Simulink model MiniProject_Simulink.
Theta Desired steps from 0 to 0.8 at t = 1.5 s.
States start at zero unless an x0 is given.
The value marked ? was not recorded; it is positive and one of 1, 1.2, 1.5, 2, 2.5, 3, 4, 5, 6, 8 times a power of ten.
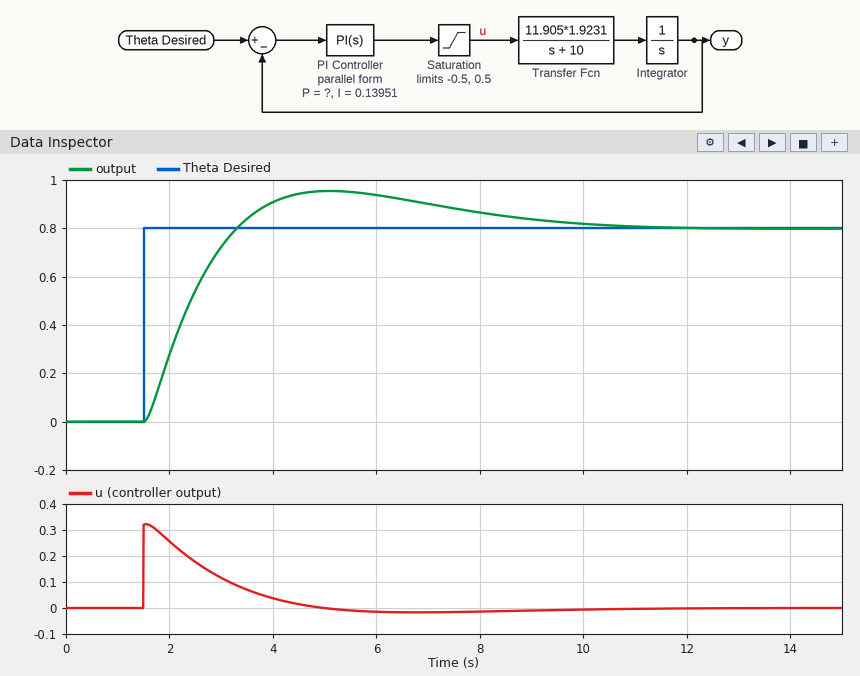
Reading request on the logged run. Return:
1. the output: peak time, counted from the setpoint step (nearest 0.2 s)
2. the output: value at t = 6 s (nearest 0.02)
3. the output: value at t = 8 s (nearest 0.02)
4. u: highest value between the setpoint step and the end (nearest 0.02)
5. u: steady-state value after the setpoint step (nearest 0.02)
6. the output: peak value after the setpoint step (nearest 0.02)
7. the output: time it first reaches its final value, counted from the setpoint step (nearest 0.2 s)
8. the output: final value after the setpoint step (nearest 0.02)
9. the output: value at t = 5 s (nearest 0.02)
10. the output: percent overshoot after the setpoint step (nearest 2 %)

3.6 s
0.94
0.86
0.32
0.00
0.96
1.8 s
0.80
0.96
20 %
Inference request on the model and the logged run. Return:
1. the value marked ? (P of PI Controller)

0.4
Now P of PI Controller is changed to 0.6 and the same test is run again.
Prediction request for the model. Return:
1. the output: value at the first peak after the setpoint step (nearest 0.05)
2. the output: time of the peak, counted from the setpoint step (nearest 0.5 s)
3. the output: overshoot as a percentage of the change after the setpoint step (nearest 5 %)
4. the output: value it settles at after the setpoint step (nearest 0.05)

0.90
3.0 s
10 %
0.80
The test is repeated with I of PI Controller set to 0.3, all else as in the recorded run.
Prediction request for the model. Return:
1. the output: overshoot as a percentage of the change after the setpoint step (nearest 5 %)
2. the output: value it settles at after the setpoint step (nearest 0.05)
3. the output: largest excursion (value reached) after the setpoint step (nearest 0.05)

30 %
0.80
1.05
